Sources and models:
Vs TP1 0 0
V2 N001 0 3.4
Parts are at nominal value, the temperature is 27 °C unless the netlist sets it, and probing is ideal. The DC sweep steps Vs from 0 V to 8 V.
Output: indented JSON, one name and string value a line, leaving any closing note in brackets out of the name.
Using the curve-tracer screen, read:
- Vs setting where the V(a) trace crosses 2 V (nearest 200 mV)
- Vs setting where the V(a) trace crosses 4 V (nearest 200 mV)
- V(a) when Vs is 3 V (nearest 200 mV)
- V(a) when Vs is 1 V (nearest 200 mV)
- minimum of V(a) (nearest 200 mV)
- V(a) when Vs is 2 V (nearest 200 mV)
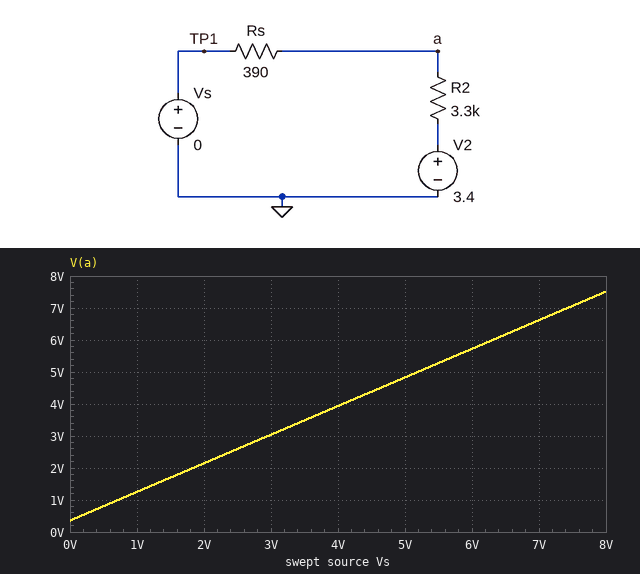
{
  "Vs setting where the V(a) trace crosses 2 V": "1.8 V",
  "Vs setting where the V(a) trace crosses 4 V": "4.0 V",
  "V(a) when Vs is 3 V": "3.0 V",
  "V(a) when Vs is 1 V": "1.2 V",
  "minimum of V(a)": "400 mV",
  "V(a) when Vs is 2 V": "2.2 V"
}
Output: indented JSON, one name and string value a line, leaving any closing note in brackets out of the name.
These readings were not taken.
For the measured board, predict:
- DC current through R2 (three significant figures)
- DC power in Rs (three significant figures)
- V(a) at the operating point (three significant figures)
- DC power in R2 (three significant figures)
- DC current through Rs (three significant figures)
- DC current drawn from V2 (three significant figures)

{
  "DC current through R2": "921 µA",
  "DC power in Rs": "331 µW",
  "V(a) at the operating point": "359 mV",
  "DC power in R2": "2.80 mW",
  "DC current through Rs": "921 µA",
  "DC current drawn from V2": "921 µA"
}
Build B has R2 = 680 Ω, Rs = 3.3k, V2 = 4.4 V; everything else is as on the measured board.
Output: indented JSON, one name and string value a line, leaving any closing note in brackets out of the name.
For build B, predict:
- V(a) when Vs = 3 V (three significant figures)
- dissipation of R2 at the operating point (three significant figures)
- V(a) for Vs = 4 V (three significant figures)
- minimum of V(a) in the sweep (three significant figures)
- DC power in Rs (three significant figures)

{
  "V(a) when Vs = 3 V": "4.16 V",
  "dissipation of R2 at the operating point": "831 µW",
  "V(a) for Vs = 4 V": "4.33 V",
  "minimum of V(a) in the sweep": "3.65 V",
  "DC power in Rs": "4.03 mW"
}
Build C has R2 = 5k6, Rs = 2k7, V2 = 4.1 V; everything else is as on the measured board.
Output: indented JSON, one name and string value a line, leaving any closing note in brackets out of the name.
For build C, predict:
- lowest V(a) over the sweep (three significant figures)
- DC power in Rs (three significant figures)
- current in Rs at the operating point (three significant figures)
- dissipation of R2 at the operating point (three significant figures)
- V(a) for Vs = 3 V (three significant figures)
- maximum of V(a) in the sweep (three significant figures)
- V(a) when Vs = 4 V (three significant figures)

{
  "lowest V(a) over the sweep": "1.33 V",
  "DC power in Rs": "659 µW",
  "current in Rs at the operating point": "494 µA",
  "dissipation of R2 at the operating point": "1.37 mW",
  "V(a) for Vs = 3 V": "3.36 V",
  "maximum of V(a) in the sweep": "6.73 V",
  "V(a) when Vs = 4 V": "4.03 V"
}
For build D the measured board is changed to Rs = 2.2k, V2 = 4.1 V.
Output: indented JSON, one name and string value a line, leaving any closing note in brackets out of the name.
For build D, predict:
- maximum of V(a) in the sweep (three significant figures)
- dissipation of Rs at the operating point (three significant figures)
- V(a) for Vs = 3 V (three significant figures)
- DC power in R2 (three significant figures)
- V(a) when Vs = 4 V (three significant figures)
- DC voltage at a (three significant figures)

{
  "maximum of V(a) in the sweep": "6.44 V",
  "dissipation of Rs at the operating point": "1.22 mW",
  "V(a) for Vs = 3 V": "3.44 V",
  "DC power in R2": "1.83 mW",
  "V(a) when Vs = 4 V": "4.04 V",
  "DC voltage at a": "1.64 V"
}
